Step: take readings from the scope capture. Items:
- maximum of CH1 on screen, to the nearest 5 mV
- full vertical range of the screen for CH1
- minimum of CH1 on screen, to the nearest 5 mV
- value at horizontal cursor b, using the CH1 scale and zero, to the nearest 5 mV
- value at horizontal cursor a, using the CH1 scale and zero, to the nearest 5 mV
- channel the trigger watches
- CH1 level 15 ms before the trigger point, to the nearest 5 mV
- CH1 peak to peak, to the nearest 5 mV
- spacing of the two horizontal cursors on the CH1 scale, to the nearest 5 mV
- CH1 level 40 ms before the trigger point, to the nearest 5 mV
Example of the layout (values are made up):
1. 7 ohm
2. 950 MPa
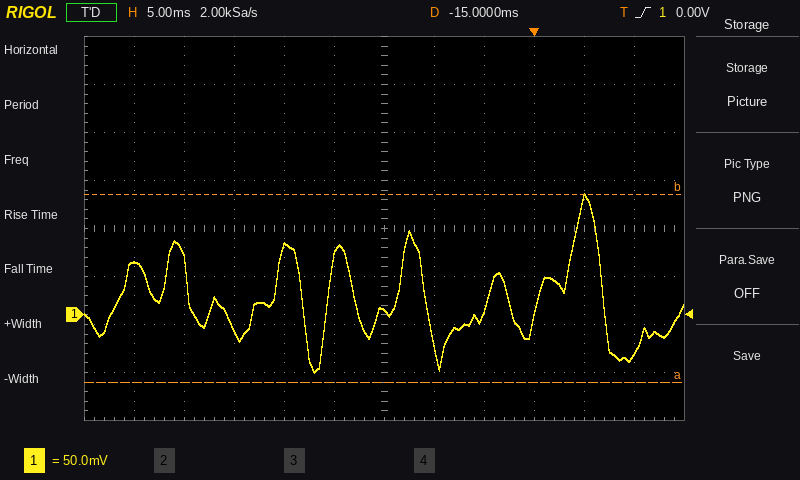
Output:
1. 125 mV
2. 400 mV
3. -60 mV
4. 125 mV
5. -70 mV
6. CH1
7. 5 mV
8. 185 mV
9. 195 mV
10. 55 mV
